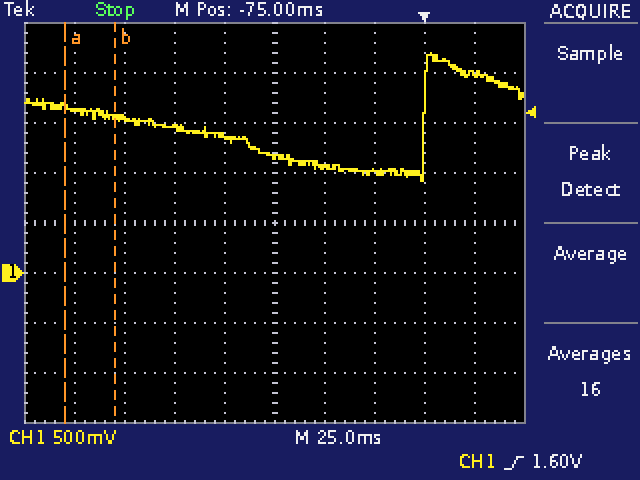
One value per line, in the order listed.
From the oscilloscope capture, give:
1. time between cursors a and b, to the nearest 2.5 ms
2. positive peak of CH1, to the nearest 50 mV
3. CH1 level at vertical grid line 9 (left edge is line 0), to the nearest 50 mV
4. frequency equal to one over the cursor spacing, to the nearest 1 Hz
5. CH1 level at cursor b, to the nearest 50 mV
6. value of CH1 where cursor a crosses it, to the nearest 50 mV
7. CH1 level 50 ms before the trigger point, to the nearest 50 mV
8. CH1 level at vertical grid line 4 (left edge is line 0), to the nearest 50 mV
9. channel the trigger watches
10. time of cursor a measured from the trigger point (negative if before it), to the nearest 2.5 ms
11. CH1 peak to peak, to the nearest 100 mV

25.0 ms
2.20 V
2.00 V
40 Hz
1.55 V
1.65 V
1.05 V
1.35 V
CH1
-180.0 ms
1.30 V
